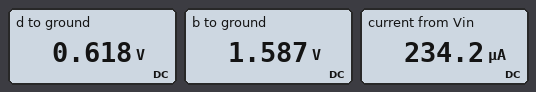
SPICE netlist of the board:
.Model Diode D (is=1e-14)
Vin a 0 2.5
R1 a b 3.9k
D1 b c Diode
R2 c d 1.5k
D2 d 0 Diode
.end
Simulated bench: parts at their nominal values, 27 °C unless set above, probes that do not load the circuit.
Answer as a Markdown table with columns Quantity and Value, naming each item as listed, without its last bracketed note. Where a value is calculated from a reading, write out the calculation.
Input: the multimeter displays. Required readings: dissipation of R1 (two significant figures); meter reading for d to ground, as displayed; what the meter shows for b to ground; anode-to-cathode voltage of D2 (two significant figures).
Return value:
| Quantity | Value |
|---|---|
| dissipation of R1 | (2.5 V - 1.587 V)^2 / 3.9 kΩ = 210 µW |
| meter reading for d to ground, as displayed | 0.618 V |
| what the meter shows for b to ground | 1.587 V |
| anode-to-cathode voltage of D2 | 618 mV = 620 mV |
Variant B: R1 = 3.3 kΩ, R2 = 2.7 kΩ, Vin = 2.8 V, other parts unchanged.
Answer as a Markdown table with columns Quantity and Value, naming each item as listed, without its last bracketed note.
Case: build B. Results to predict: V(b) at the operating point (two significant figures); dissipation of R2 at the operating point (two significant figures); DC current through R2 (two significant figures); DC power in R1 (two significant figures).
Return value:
| Quantity | Value |
|---|---|
| V(b) at the operating point | 1.9 V |
| dissipation of R2 at the operating point | 180 µW |
| DC current through R2 | 260 µA |
| DC power in R1 | 220 µW |
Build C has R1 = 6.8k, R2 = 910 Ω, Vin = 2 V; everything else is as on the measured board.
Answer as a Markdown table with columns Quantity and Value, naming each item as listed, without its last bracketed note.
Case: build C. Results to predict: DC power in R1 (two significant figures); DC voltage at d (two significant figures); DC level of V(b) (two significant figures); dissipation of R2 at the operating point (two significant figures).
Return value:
| Quantity | Value |
|---|---|
| DC power in R1 | 74 µW |
| DC voltage at d | 600 mV |
| DC level of V(b) | 1.3 V |
| dissipation of R2 at the operating point | 10 µW |
